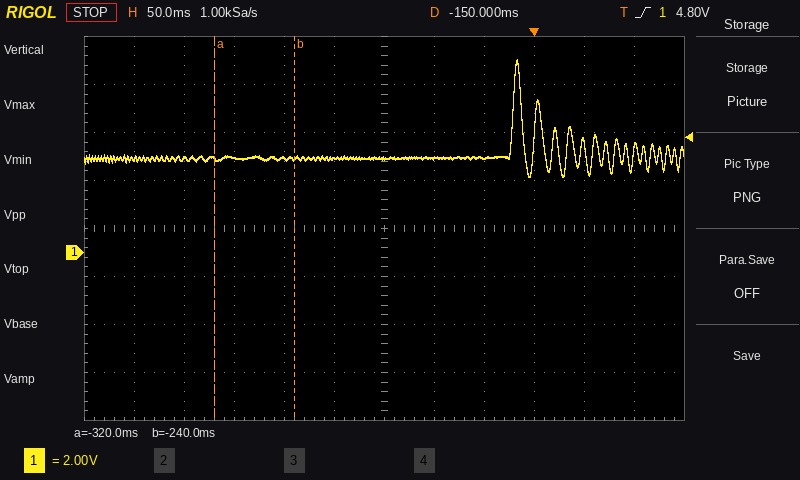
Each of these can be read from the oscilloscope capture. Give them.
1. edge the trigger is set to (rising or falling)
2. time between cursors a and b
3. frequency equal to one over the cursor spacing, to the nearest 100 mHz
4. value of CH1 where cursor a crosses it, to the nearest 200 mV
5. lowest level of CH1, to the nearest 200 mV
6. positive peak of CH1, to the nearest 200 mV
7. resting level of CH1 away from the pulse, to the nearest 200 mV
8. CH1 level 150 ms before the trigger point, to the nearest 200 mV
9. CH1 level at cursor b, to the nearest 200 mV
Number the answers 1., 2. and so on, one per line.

1. rising
2. 80 ms
3. 12.5 Hz
4. 4.0 V
5. 3.2 V
6. 8.0 V
7. 4.0 V
8. 4.0 V
9. 4.0 V
